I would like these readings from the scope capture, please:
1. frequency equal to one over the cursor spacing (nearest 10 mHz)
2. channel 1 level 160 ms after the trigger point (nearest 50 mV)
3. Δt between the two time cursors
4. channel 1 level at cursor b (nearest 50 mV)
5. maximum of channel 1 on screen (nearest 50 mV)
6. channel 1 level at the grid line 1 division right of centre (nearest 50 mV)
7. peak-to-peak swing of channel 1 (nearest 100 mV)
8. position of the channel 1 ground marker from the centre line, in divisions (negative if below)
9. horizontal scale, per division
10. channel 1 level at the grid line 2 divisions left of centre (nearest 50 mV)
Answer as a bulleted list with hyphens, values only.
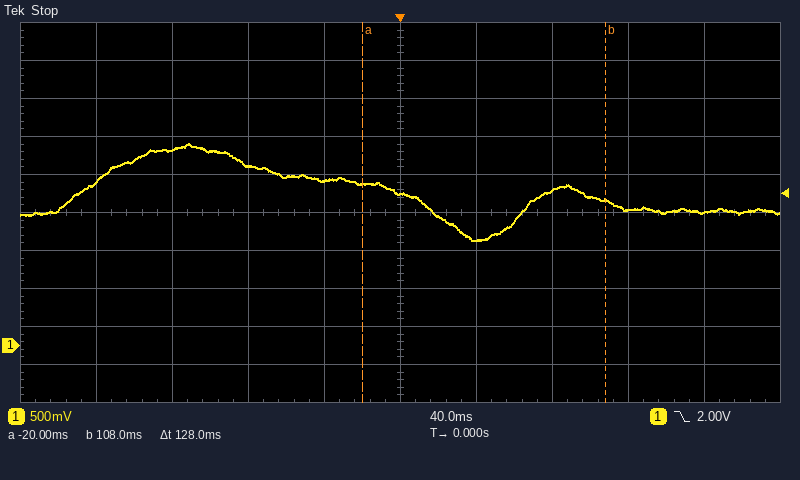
- 7.81 Hz
- 1.75 V
- 128 ms
- 1.90 V
- 2.65 V
- 1.40 V
- 1.30 V
- -3.5 div
- 40 ms
- 2.35 V
